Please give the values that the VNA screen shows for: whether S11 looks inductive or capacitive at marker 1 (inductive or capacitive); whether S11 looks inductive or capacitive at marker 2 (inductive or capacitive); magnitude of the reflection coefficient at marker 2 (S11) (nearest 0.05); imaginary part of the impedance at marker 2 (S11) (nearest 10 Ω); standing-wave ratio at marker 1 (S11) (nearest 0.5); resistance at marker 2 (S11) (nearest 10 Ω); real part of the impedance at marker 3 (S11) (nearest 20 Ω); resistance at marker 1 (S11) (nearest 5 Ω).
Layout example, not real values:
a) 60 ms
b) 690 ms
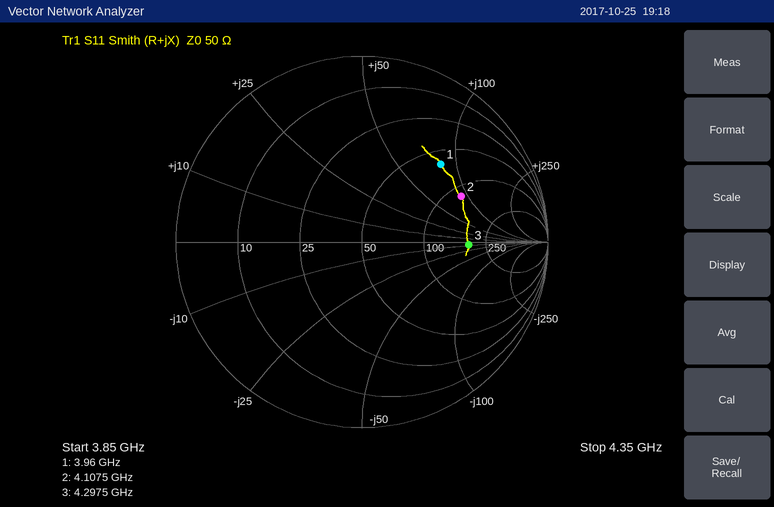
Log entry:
a) inductive
b) inductive
c) 0.60
d) +90 Ω
e) 4.0
f) 120 Ω
g) 180 Ω
h) 65 Ω
